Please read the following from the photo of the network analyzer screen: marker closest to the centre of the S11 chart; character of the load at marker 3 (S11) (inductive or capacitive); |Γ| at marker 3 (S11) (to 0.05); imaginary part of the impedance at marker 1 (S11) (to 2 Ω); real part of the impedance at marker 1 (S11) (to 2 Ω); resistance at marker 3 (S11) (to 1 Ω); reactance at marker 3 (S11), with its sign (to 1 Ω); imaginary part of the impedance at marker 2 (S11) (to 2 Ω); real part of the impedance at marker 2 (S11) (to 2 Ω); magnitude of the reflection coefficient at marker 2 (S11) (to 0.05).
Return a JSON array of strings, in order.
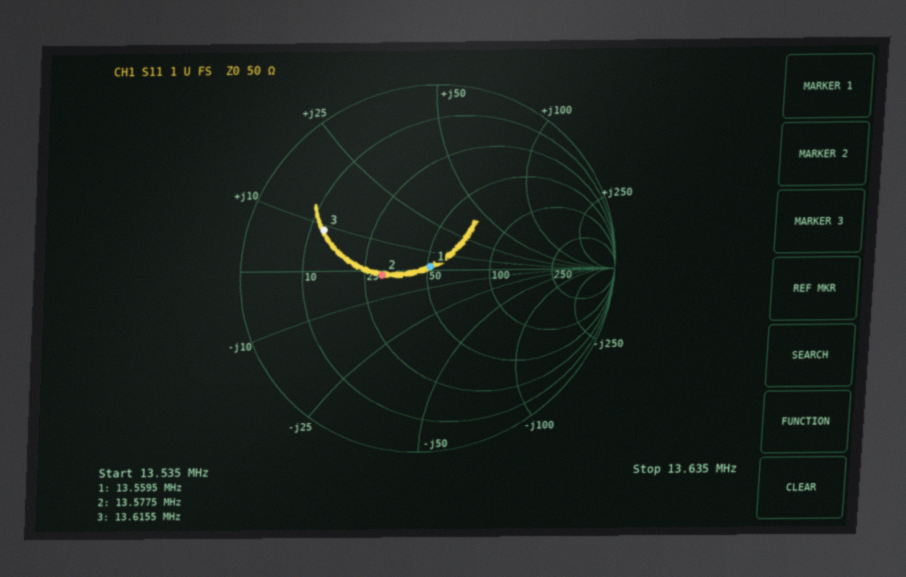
["marker 1", "inductive", "0.60", "+2 Ω", "52 Ω", "13 Ω", "+9 Ω", "-2 Ω", "30 Ω", "0.25"]
